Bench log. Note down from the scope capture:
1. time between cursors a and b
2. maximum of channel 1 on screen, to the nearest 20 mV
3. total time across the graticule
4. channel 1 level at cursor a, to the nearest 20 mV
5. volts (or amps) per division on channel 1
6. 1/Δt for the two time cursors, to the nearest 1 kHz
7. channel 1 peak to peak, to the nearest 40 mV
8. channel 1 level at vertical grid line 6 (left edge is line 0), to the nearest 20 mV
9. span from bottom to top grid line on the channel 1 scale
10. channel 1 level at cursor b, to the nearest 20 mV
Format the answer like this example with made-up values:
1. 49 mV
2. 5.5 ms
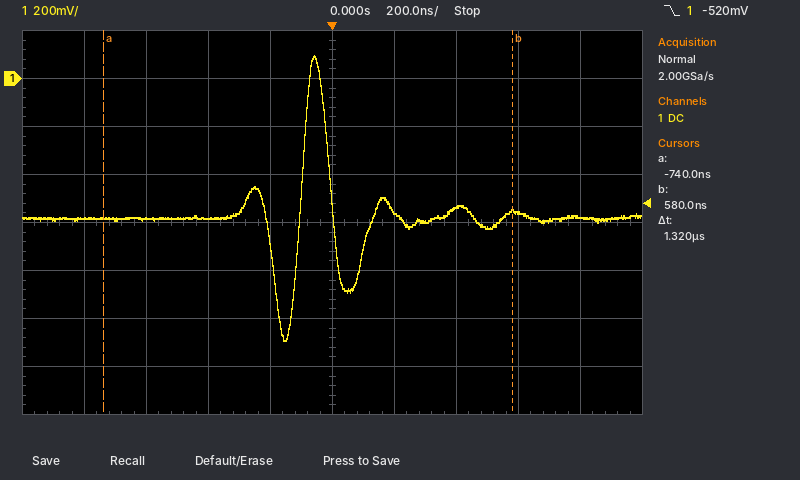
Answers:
1. 1.32 µs
2. 100 mV
3. 2 µs
4. -580 mV
5. 200 mV
6. 758 kHz
7. 1.20 V
8. -560 mV
9. 1.6 V
10. -560 mV
